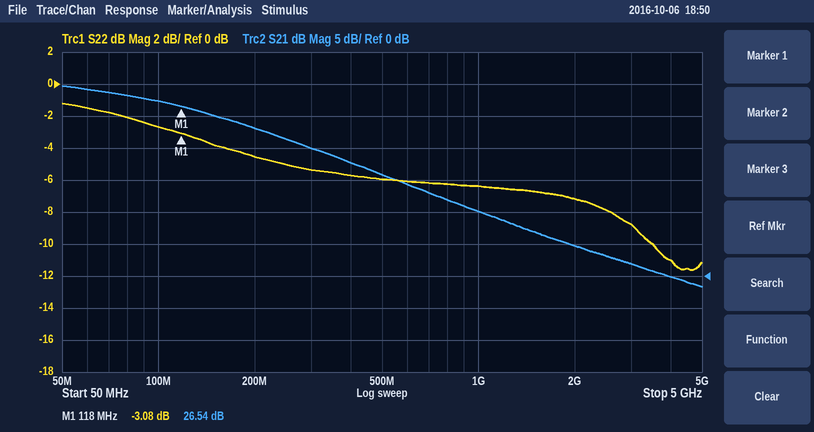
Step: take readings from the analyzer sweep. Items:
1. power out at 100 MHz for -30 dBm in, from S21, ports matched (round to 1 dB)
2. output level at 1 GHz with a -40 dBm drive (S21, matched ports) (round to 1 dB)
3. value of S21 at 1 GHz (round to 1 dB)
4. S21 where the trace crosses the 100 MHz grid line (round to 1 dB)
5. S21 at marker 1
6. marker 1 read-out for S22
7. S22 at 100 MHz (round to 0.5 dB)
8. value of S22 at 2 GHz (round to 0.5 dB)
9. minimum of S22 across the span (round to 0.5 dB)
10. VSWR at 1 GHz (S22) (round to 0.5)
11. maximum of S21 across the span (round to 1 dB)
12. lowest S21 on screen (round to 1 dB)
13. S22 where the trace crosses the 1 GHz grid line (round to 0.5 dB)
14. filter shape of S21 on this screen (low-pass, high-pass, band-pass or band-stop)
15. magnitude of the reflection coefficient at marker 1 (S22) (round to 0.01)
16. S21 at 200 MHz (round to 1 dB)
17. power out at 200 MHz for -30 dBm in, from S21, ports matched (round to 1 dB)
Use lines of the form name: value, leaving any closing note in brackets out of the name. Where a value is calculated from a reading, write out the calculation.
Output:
power out at 100 MHz for -30 dBm in, from S21, ports matched: -30 dBm + (27 dB) = -3 dBm
output level at 1 GHz with a -40 dBm drive (S21, matched ports): -40 dBm + (10 dB) = -30 dBm
value of S21 at 1 GHz: 10 dB
S21 where the trace crosses the 100 MHz grid line: 27 dB
S21 at marker 1: 26.54 dB
marker 1 read-out for S22: -3.08 dB
S22 at 100 MHz: -2.5 dB
value of S22 at 2 GHz: -7.0 dB
minimum of S22 across the span: -11.5 dB
VSWR at 1 GHz (S22): |Γ| = 10^(-6.5/20) = 0.4732; VSWR = (1 + 0.4732)/(1 − 0.4732) ≈ 2.80, so 3.0 to the nearest 0.5
maximum of S21 across the span: 30 dB
lowest S21 on screen: -2 dB
S22 where the trace crosses the 1 GHz grid line: -6.5 dB
filter shape of S21 on this screen: low-pass
magnitude of the reflection coefficient at marker 1 (S22): 10^(-3.08/20) ≈ 0.70
S21 at 200 MHz: 23 dB
power out at 200 MHz for -30 dBm in, from S21, ports matched: -30 dBm + (23 dB) = -7 dBm
